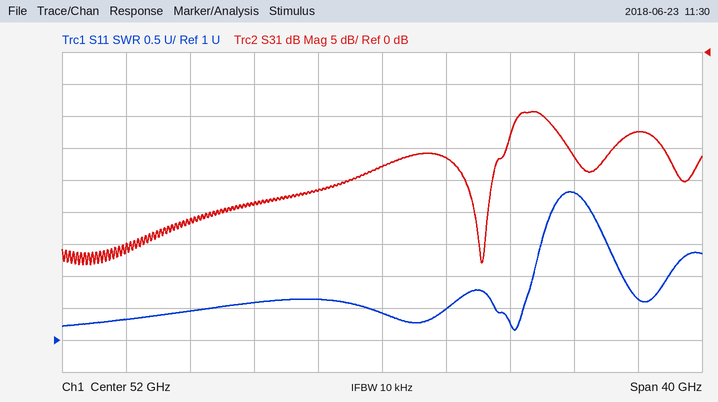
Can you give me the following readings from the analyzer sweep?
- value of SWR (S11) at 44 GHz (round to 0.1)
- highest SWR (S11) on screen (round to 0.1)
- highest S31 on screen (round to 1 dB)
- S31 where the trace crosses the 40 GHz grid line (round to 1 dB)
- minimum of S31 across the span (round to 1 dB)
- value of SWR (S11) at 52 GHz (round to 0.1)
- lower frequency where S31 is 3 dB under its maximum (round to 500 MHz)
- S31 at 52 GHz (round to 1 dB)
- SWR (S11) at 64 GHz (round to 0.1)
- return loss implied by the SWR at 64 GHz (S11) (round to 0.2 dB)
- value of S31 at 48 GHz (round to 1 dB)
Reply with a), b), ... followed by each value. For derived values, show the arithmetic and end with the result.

a) 1.6
b) 3.3
c) -9 dB
d) -26 dB
e) -33 dB
f) 1.4
g) 60.0 GHz
h) -18 dB
i) 3.3
j) −20 log10((3.3 − 1)/(3.3 + 1)) ≈ 5.4 dB
k) -22 dB
